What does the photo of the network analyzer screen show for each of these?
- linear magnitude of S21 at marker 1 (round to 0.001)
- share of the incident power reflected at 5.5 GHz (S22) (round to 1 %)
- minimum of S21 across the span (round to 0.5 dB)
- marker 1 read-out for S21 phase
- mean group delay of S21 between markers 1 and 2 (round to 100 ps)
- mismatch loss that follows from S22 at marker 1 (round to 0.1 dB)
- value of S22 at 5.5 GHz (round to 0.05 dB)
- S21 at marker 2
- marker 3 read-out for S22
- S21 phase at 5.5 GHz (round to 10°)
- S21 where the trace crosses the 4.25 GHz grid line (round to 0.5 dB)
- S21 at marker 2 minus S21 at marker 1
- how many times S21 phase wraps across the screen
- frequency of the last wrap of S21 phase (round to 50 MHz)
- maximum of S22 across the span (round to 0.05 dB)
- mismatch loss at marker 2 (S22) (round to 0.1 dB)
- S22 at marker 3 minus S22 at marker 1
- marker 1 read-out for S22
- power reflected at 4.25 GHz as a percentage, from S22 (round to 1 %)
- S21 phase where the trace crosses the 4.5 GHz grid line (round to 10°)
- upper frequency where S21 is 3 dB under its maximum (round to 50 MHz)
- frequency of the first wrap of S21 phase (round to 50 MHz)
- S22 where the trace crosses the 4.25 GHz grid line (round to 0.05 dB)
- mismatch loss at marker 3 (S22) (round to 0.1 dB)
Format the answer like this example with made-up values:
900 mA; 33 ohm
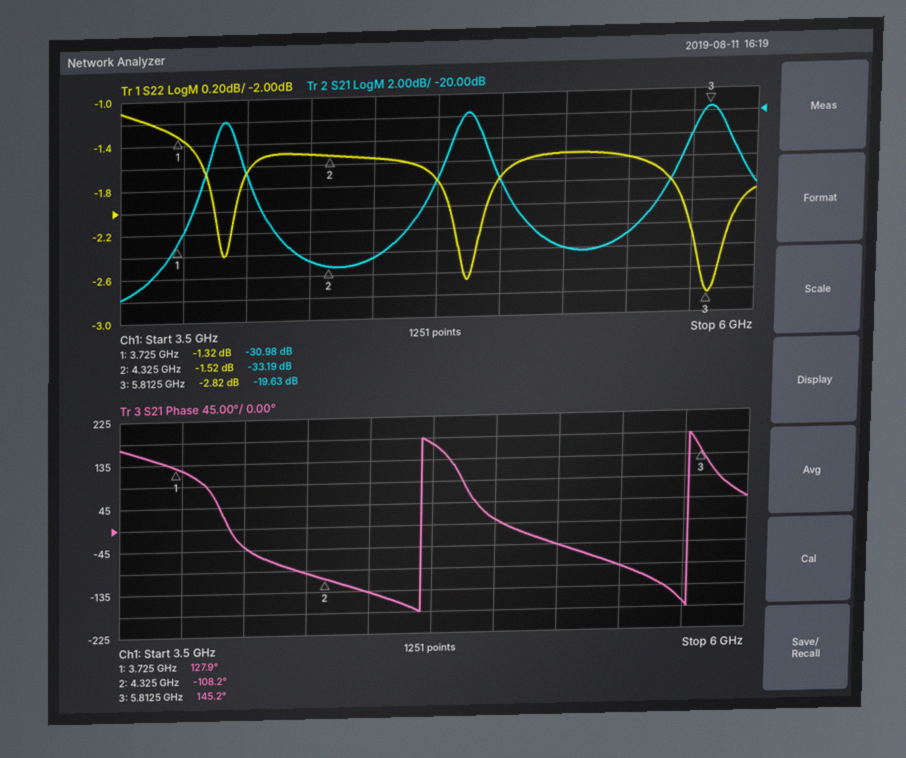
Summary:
0.028; 69 %; -36.0 dB; 127.9°; 1.1 ns; 5.8 dB; -1.60 dB; -33.19 dB; -2.82 dB; -90°; -32.5 dB; -2.21 dB; 2; 5.75 GHz; -1.10 dB; 5.3 dB; -1.50 dB; -1.32 dB; 71 %; -140°; 5.90 GHz; 4.70 GHz; -1.50 dB; 3.2 dB
